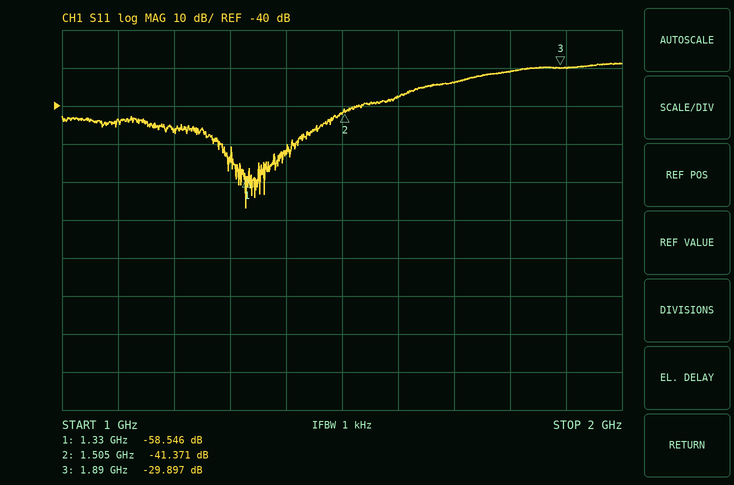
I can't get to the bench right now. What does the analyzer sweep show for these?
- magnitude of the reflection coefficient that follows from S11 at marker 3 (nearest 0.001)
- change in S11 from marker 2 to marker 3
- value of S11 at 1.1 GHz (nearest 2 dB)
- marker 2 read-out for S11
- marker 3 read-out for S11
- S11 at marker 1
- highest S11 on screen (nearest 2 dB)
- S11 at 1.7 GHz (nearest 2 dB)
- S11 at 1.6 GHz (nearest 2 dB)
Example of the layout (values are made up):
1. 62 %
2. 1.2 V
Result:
1. 0.032
2. 11.474 dB
3. -44 dB
4. -41.371 dB
5. -29.897 dB
6. -58.546 dB
7. -28 dB
8. -34 dB
9. -38 dB
